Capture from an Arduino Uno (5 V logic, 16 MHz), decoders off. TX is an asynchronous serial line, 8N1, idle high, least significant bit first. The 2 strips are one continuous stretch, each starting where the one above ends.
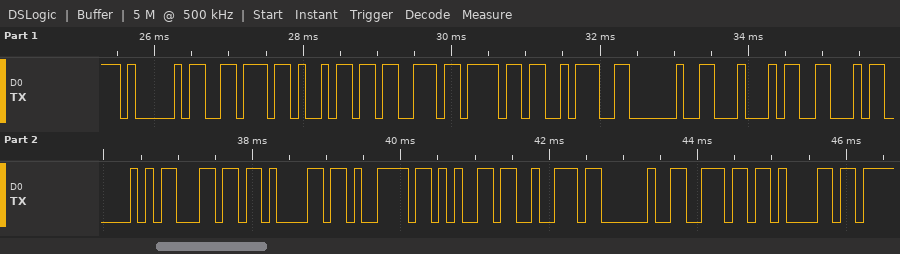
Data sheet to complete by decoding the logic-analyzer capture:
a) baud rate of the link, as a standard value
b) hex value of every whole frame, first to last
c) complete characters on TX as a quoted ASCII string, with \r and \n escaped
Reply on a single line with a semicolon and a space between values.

9600 baud; 41 76 69 73 6F 3A 20 44 46 50 6C 61 79 65 72 20 6E 61; "Aviso: DFPlayer na"
